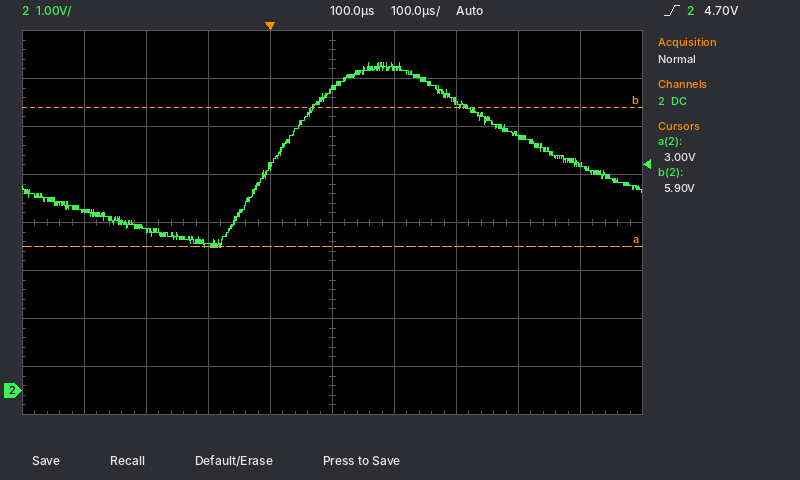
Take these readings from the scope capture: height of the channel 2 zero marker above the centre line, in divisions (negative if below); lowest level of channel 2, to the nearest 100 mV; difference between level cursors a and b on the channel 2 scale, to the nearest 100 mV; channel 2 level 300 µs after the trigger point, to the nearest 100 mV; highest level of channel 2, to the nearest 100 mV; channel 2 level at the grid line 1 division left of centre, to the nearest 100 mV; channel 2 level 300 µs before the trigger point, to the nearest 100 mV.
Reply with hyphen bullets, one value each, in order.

- -3.5 div
- 3.0 V
- 2.9 V
- 6.0 V
- 6.8 V
- 4.7 V
- 3.7 V
